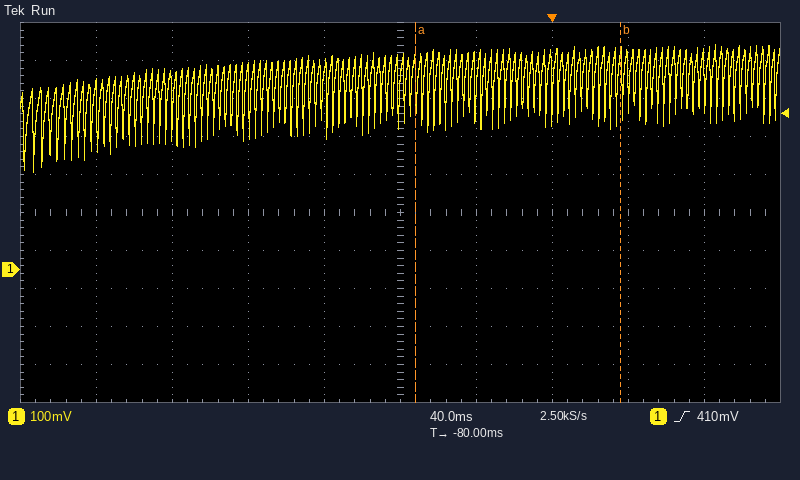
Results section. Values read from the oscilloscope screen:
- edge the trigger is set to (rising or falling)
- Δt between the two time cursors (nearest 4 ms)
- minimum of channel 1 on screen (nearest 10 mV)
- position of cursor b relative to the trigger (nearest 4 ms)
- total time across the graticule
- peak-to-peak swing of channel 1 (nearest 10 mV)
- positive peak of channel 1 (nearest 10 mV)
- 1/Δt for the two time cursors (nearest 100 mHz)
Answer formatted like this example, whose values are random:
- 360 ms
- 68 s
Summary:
- rising
- 108 ms
- 260 mV
- +36 ms
- 400 ms
- 330 mV
- 590 mV
- 9.3 Hz
